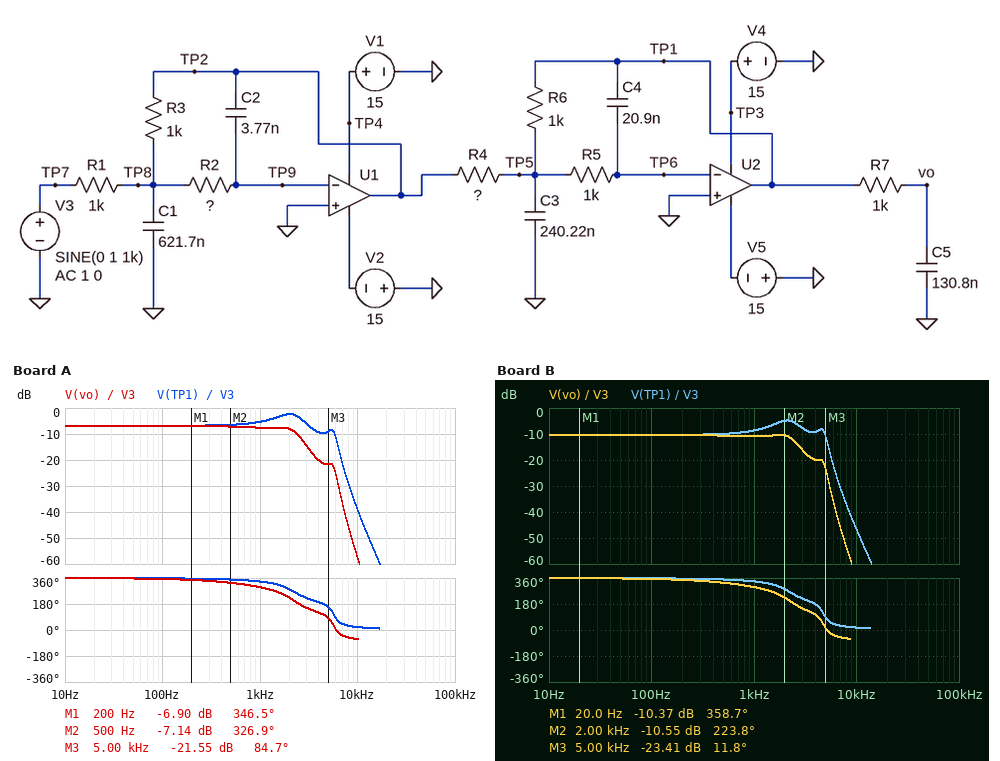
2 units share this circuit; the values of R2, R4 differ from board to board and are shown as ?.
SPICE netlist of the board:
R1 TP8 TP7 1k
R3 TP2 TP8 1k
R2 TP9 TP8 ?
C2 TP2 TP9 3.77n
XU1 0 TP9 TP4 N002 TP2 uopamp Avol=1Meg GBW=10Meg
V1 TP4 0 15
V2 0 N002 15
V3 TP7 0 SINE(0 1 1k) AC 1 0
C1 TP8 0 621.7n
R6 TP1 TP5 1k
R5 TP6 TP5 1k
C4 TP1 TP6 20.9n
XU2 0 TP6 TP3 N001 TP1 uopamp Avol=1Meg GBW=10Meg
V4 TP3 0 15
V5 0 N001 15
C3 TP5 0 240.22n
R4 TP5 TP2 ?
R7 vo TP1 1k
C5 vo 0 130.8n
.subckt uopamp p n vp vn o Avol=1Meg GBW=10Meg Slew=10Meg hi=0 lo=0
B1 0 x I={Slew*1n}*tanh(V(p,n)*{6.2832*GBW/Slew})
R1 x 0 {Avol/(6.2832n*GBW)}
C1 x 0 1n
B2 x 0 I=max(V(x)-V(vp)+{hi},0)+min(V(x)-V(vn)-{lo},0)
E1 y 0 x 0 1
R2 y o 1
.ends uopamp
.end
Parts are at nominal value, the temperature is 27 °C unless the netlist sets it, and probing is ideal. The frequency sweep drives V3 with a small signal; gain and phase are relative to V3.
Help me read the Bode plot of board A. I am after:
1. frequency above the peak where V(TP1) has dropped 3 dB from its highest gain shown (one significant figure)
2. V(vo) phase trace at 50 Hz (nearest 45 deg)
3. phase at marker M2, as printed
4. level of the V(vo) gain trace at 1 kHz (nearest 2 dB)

3 kHz
360 deg
326.9 deg
-8 dB
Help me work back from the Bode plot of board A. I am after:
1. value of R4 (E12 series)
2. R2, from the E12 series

2.2 kΩ
330 Ω
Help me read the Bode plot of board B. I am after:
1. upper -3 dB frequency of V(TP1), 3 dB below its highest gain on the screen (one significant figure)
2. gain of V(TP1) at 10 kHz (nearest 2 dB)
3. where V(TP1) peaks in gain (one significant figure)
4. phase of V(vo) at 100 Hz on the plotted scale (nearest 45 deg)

3 kHz
-46 dB
2 kHz
360 deg
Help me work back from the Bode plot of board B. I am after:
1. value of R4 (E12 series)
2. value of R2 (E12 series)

3.3 kΩ
470 Ω
